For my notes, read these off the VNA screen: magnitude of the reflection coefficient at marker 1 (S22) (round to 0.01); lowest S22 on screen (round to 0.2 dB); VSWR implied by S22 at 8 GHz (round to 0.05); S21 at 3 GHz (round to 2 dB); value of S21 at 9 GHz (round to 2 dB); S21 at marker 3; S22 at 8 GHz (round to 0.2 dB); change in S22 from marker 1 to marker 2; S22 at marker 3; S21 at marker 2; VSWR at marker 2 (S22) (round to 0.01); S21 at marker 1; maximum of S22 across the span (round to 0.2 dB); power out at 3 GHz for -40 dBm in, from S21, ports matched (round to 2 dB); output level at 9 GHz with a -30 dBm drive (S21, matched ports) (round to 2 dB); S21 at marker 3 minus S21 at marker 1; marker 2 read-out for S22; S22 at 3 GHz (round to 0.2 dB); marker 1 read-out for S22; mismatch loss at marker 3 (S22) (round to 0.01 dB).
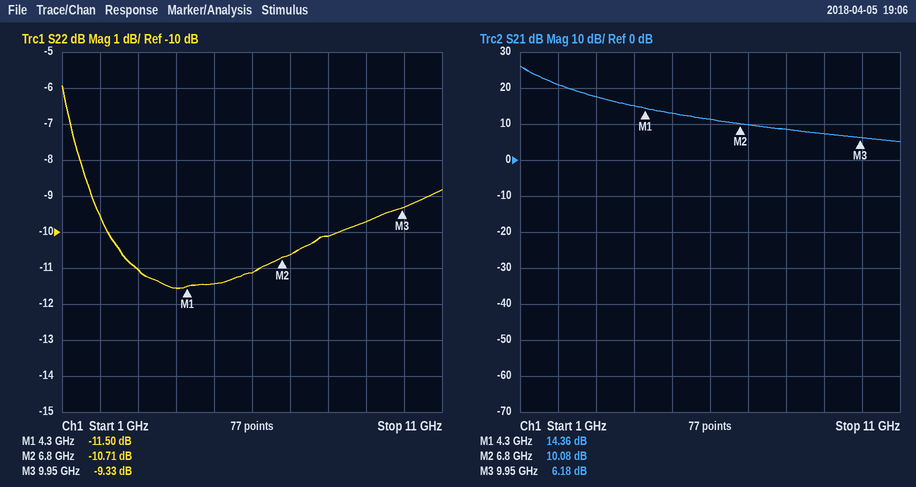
0.27
-11.6 dB
1.90
18 dB
8 dB
6.18 dB
-10.2 dB
0.79 dB
-9.33 dB
10.08 dB
1.82
14.36 dB
-6.0 dB
-22 dBm
-22 dBm
-8.18 dB
-10.71 dB
-11.0 dB
-11.50 dB
0.54 dB
